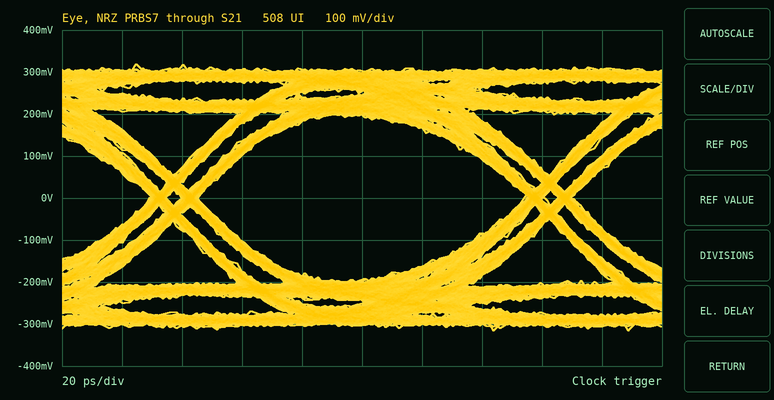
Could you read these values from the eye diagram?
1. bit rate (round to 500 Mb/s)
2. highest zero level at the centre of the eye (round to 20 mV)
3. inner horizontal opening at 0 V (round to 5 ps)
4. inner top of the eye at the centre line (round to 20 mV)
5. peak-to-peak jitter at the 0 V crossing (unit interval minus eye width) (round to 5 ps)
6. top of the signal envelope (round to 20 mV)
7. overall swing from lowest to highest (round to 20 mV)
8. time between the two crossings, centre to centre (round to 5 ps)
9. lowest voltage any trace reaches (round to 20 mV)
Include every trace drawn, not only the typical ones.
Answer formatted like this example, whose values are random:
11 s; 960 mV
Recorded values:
8.0 Gb/s; -200 mV; 110 ps; 200 mV; 15 ps; 320 mV; 640 mV; 125 ps; -320 mV
